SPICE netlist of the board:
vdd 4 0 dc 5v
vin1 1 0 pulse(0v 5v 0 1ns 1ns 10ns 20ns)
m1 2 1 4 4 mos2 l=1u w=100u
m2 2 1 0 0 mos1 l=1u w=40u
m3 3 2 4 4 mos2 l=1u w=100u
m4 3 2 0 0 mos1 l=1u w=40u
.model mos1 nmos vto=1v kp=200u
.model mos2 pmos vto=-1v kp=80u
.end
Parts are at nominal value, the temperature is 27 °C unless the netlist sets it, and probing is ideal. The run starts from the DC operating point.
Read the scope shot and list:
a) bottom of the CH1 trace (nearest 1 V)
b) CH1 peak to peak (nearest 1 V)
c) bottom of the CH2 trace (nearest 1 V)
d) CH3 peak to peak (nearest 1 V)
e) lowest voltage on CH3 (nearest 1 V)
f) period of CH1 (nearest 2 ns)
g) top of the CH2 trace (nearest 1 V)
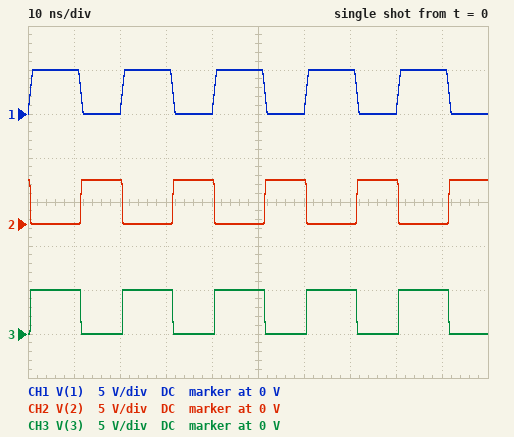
0 V
5 V
0 V
5 V
0 V
20 ns
5 V
